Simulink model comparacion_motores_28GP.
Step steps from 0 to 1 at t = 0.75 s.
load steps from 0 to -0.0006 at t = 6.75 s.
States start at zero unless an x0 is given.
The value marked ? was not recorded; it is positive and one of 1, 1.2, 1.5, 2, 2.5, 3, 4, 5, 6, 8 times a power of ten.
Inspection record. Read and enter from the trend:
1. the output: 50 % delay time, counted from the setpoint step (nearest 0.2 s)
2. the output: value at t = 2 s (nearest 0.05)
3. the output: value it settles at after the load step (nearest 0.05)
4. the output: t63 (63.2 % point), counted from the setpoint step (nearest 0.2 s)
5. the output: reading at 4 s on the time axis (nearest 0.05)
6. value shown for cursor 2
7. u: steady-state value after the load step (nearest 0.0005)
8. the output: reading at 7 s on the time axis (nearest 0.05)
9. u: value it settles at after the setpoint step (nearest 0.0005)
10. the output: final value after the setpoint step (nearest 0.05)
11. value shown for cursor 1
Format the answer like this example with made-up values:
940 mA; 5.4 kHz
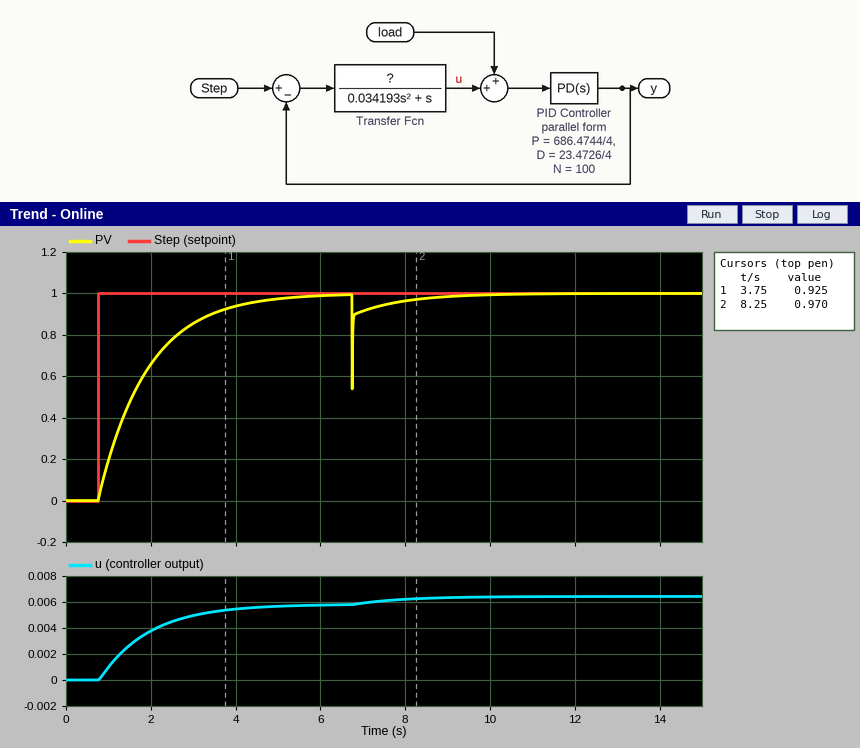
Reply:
0.8 s; 0.65; 1.00; 1.2 s; 0.95; 0.970; 0.0065; 0.90; 0.0060; 1.00; 0.925
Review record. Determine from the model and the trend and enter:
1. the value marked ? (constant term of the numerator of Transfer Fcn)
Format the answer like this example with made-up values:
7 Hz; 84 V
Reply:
0.005
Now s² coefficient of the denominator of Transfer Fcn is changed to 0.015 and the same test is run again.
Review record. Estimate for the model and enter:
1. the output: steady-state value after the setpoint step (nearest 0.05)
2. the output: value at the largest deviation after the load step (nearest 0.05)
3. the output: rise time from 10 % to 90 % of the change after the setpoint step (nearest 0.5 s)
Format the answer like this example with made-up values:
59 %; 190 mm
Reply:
1.00; 0.55; 2.5 s
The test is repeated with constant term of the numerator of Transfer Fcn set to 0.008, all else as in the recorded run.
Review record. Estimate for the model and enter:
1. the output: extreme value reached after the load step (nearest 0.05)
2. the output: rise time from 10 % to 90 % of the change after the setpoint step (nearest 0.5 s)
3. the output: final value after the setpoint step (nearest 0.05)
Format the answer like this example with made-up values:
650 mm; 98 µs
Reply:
0.55; 1.5 s; 1.00
